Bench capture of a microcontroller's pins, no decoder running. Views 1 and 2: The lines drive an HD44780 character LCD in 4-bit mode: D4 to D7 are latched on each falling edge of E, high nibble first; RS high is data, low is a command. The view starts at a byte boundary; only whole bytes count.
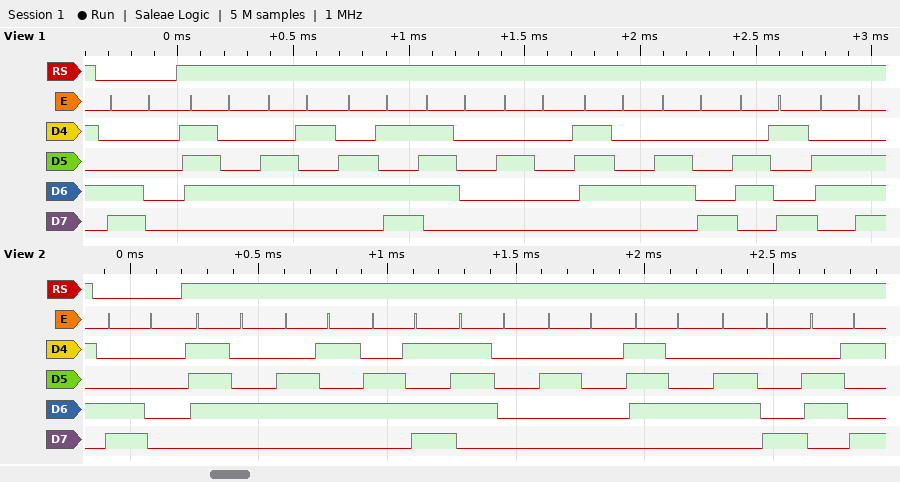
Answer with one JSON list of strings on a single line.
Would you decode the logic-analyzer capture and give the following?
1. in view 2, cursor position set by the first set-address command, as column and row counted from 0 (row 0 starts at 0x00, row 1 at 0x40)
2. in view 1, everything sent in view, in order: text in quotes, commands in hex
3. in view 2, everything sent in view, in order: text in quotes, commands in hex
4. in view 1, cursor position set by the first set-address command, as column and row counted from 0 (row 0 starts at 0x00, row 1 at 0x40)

["column 0, row 1", "0xC0 \"temp thin\"", "0xC0 \"temp thi\"", "column 0, row 1"]
